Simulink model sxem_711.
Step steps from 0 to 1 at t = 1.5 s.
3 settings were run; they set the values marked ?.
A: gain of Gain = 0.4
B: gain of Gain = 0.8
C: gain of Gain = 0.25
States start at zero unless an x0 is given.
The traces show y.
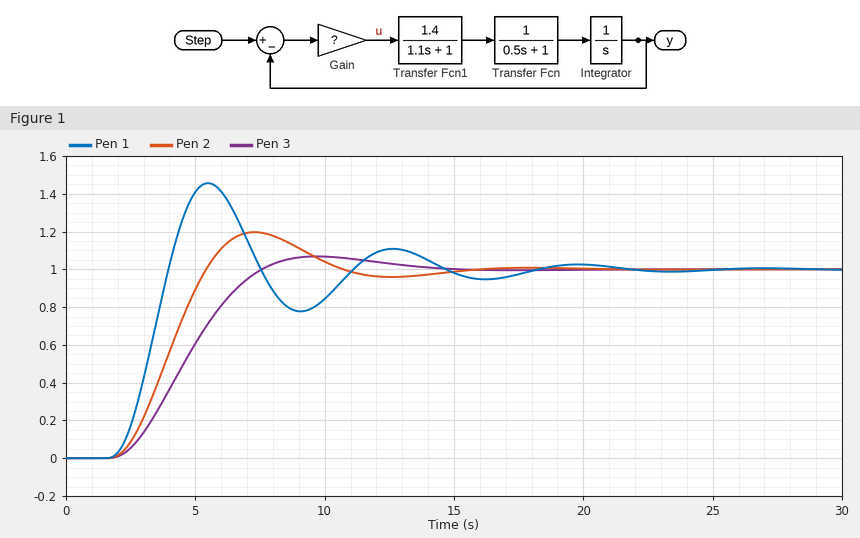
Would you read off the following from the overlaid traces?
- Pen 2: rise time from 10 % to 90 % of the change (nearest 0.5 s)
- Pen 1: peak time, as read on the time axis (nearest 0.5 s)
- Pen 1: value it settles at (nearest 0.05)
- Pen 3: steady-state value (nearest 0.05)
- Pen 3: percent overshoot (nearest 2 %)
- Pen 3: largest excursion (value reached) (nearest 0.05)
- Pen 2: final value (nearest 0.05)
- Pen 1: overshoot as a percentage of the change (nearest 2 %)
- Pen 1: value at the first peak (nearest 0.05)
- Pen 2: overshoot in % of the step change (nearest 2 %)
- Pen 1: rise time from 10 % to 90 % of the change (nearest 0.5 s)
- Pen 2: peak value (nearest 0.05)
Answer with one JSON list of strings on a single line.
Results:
["2.5 s", "5.5 s", "1.00", "1.00", "6 %", "1.05", "1.00", "46 %", "1.45", "20 %", "1.5 s", "1.20"]
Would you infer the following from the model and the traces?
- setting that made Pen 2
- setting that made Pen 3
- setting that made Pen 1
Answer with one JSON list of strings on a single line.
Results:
["A", "C", "B"]
